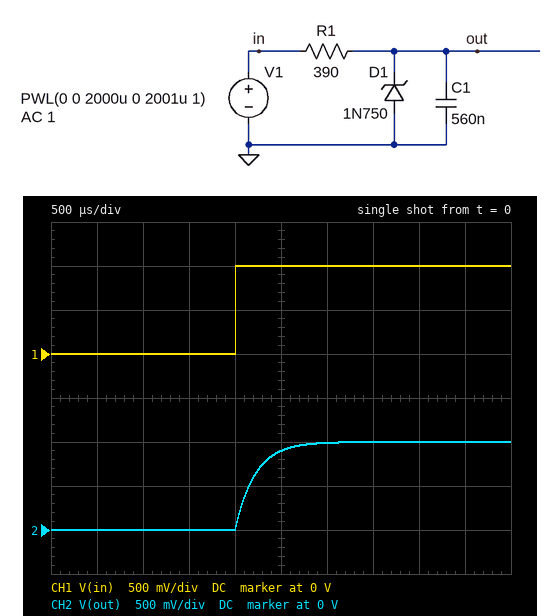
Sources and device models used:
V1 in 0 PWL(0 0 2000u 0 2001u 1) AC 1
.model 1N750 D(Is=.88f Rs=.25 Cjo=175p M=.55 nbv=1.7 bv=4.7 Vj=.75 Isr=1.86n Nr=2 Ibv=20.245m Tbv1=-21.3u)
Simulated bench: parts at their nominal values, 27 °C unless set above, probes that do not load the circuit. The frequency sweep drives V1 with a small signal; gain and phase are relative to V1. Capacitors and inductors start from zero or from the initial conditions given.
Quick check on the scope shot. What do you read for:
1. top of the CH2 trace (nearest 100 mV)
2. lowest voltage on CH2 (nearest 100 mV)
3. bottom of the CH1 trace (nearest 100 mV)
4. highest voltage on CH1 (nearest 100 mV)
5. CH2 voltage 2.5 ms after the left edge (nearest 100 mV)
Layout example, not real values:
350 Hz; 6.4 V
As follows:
1.0 V; 0 V; 0 V; 1.0 V; 900 mV
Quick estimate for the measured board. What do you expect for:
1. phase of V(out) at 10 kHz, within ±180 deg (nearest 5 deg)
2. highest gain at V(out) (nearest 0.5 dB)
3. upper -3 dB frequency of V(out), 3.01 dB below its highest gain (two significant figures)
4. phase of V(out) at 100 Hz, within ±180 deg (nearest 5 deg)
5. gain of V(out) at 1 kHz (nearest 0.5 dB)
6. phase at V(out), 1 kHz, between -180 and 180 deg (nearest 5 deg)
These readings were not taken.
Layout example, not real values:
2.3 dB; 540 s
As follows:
-85 deg; 0 dB; 730 Hz; -10 deg; -4.5 dB; -55 deg
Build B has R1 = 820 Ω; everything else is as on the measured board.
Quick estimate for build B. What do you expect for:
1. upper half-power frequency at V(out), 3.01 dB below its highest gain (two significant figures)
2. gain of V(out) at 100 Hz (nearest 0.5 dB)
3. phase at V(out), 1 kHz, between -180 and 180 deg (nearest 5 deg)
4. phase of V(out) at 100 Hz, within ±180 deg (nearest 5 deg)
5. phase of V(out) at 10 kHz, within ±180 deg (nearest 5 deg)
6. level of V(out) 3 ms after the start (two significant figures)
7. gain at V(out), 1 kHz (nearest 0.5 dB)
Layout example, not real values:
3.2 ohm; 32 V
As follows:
350 Hz; -0.5 dB; -70 deg; -15 deg; -90 deg; 890 mV; -9.5 dB
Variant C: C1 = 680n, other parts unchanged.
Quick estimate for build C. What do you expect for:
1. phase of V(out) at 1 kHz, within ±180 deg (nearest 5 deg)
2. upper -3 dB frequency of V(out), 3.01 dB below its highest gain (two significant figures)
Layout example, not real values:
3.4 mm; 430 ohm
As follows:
-60 deg; 600 Hz
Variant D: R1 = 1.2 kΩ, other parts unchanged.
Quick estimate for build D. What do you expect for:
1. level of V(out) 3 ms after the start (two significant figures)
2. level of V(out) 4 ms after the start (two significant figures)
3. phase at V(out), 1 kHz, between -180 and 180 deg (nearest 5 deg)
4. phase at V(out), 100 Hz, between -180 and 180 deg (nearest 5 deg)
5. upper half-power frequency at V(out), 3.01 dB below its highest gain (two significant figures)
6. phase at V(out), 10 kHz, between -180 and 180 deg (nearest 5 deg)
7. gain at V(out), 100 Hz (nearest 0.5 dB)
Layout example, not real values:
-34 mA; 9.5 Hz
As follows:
770 mV; 950 mV; -75 deg; -25 deg; 240 Hz; -90 deg; -0.5 dB
